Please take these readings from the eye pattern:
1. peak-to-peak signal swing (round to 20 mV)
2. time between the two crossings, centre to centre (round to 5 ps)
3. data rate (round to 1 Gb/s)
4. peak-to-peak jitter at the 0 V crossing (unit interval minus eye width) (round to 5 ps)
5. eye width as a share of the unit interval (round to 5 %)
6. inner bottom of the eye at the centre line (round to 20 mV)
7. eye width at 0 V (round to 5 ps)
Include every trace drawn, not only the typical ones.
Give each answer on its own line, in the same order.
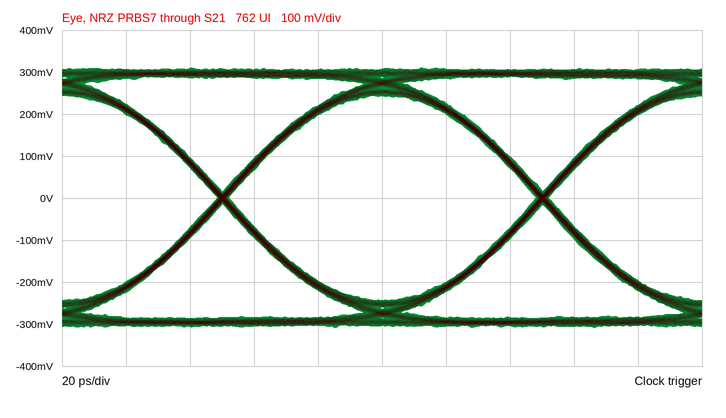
620 mV
100 ps
10 Gb/s
5 ps
95 %
-240 mV
95 ps
